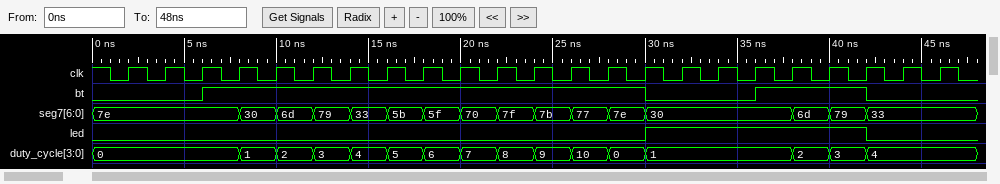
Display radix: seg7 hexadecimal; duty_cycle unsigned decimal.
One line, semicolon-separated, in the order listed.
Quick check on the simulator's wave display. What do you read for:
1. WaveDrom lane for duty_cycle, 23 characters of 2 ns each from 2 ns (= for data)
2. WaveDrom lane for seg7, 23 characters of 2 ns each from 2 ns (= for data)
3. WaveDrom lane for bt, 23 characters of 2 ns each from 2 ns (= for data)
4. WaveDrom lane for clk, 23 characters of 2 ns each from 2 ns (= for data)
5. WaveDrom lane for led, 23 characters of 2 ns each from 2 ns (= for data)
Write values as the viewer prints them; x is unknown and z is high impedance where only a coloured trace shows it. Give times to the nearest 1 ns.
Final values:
{name: 'duty_cycle', wave: '=..============...===..', data: '0 1 2 3 4 5 6 7 8 9 10 0 1 2 3 4'}; {name: 'seg7', wave: '=..============...===..', data: '7e 30 6d 79 33 5b 5f 70 7f 7b 77 7e 30 6d 79 33'}; {name: 'bt', wave: '0.1...........0..1..0..'}; {name: 'clk', wave: 'p......................'}; {name: 'led', wave: '0.............1.....0..'}
